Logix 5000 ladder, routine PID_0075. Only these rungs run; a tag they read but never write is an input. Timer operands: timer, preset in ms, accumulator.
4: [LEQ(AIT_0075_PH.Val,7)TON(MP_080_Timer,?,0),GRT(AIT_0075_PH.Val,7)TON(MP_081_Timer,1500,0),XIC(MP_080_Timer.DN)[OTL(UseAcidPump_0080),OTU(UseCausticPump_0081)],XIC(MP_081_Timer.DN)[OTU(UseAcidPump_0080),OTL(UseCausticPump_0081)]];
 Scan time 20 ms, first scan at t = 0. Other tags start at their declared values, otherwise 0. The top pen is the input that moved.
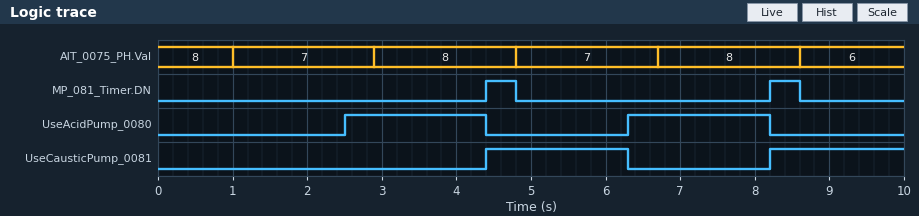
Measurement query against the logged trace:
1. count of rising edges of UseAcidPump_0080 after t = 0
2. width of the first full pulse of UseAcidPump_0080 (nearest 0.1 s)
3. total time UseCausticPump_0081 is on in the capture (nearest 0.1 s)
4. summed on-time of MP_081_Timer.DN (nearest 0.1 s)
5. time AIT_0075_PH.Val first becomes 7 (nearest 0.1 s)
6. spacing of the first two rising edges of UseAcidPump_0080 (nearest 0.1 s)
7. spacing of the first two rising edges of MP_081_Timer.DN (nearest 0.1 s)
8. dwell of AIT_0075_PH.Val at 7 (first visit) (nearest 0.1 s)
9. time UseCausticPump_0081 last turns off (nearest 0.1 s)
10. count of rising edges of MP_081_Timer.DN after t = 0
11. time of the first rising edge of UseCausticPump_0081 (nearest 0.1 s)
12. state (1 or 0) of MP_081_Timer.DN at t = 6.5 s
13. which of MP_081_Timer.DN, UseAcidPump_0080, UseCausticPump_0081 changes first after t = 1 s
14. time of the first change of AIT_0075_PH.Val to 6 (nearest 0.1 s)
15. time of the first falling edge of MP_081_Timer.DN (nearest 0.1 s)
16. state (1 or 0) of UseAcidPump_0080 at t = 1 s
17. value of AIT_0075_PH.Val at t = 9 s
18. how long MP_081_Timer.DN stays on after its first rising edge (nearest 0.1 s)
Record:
2
1.9 s
3.7 s
0.8 s
1.0 s
3.8 s
3.8 s
1.9 s
6.3 s
2
4.4 s
0
UseAcidPump_0080
8.6 s
4.8 s
0
6
0.4 s
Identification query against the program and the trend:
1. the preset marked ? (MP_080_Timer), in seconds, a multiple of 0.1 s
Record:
1.5 s
